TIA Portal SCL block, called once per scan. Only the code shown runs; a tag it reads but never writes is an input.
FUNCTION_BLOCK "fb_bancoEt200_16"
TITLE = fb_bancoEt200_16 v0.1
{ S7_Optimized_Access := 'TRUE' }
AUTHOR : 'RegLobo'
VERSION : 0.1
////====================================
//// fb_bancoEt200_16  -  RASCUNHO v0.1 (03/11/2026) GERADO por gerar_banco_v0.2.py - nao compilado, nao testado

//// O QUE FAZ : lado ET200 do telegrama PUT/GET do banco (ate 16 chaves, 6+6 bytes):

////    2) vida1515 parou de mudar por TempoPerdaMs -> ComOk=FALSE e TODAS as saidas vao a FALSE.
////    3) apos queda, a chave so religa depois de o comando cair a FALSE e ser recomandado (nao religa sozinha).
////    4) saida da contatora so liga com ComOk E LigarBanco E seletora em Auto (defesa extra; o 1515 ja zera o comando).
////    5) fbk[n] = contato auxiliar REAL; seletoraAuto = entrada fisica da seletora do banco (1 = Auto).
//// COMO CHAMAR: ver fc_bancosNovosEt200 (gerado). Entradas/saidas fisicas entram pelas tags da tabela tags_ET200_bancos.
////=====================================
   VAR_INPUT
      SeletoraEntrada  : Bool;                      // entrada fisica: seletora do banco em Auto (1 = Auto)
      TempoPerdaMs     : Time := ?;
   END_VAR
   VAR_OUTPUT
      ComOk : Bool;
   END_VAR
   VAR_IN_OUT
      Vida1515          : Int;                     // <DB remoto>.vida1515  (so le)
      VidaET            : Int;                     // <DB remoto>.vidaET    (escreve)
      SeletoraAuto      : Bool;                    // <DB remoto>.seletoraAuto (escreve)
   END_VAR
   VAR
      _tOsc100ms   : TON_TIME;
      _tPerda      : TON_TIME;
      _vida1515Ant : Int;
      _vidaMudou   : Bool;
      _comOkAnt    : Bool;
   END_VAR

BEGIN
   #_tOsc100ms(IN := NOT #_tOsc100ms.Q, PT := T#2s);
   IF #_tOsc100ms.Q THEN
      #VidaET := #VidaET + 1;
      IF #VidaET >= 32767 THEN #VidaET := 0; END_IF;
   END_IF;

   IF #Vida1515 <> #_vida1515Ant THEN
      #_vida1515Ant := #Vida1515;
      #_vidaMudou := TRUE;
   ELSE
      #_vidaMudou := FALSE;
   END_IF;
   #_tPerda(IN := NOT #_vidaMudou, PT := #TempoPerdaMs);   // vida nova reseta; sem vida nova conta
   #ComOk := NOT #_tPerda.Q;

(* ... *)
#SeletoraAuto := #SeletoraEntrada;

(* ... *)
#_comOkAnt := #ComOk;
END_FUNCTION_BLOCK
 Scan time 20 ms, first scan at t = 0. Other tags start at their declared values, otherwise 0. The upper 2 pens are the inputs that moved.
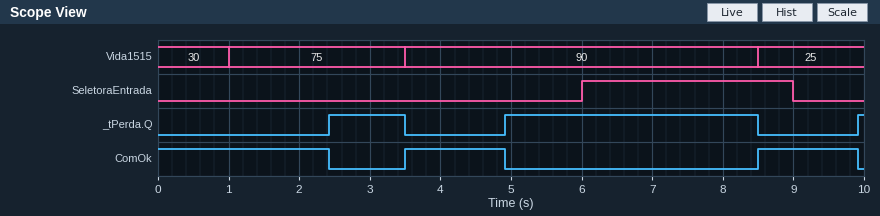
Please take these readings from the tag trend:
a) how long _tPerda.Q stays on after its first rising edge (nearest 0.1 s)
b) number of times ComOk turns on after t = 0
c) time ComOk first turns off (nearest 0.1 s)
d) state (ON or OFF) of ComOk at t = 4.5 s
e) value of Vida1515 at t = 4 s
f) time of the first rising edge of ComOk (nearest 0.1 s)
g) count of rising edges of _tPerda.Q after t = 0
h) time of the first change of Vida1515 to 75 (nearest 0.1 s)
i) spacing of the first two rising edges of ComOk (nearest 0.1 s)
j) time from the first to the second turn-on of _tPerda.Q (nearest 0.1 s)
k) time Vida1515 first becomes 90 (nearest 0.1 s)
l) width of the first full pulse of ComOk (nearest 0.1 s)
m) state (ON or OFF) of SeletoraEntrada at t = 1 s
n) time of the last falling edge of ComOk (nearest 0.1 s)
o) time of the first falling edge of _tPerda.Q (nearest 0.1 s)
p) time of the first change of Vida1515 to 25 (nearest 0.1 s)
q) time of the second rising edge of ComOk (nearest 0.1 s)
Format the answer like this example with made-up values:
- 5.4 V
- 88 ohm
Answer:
- 1.1 s
- 2
- 2.4 s
- ON
- 90
- 3.5 s
- 3
- 1.0 s
- 5.0 s
- 2.5 s
- 3.5 s
- 1.4 s
- OFF
- 9.9 s
- 3.5 s
- 8.5 s
- 8.5 s
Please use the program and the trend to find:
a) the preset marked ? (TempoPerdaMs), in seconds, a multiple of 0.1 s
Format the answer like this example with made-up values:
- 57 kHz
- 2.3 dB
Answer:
- 1.4 s
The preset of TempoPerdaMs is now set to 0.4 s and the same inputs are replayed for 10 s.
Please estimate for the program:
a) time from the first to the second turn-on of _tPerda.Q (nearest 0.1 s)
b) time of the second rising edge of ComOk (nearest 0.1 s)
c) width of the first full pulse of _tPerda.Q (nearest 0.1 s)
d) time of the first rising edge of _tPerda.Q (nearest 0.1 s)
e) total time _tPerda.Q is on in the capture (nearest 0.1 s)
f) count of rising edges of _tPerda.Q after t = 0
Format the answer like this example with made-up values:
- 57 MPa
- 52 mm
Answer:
- 1.0 s
- 3.5 s
- 0.6 s
- 0.4 s
- 8.3 s
- 4
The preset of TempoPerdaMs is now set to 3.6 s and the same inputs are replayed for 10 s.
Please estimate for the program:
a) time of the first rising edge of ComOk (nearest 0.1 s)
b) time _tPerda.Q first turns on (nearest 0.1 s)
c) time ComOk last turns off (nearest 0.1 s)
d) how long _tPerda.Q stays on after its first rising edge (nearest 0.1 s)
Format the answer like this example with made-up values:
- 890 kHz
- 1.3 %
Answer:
- 8.5 s
- 7.1 s
- 7.1 s
- 1.4 s
